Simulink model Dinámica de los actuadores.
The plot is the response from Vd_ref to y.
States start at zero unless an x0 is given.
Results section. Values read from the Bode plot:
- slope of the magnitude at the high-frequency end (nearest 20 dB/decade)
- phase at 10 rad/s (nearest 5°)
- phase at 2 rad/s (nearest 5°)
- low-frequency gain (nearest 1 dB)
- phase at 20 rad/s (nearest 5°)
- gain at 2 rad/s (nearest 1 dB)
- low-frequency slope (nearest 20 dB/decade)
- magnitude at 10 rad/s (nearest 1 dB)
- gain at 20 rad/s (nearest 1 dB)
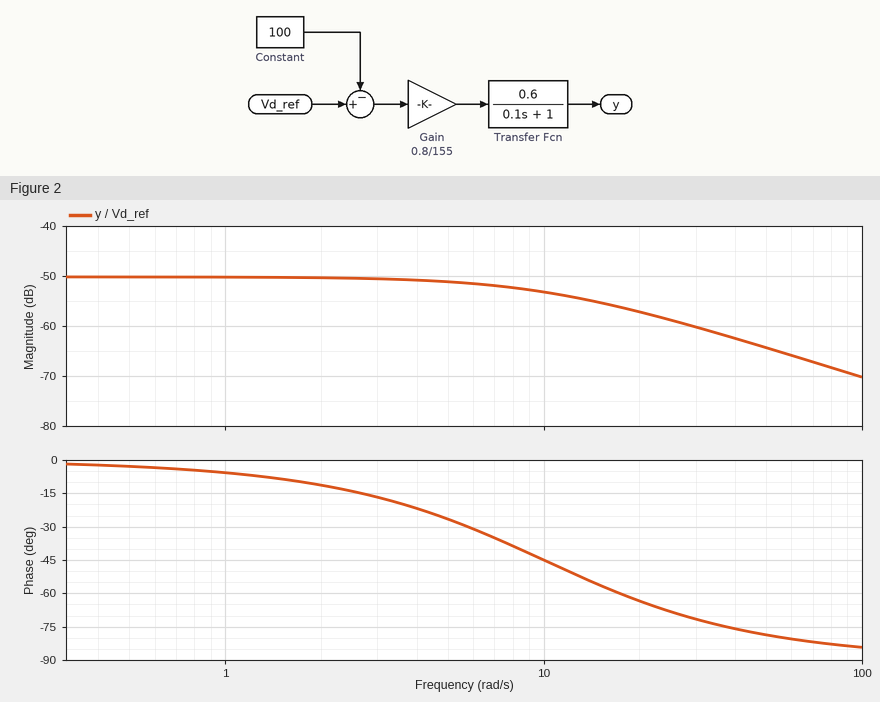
-20 dB/decade
-45°
-10°
-50 dB
-65°
-50 dB
0 dB/decade
-53 dB
-57 dB
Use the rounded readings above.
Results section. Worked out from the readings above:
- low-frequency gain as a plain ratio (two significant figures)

0.0032
